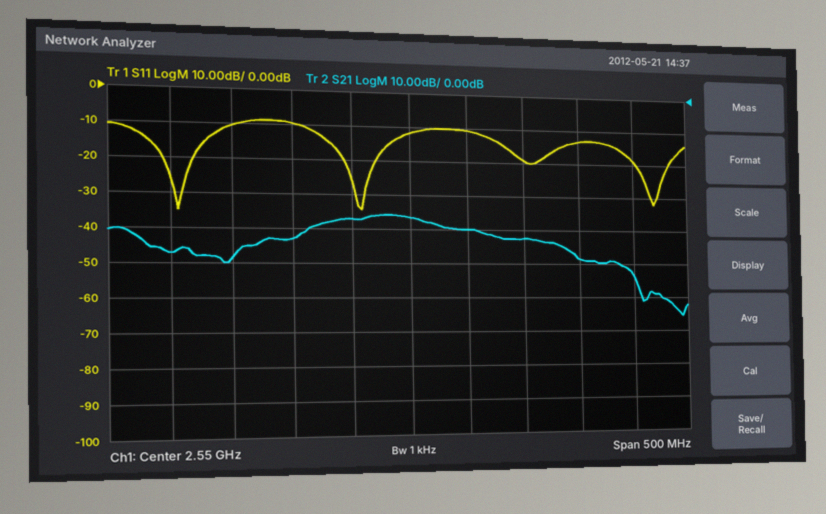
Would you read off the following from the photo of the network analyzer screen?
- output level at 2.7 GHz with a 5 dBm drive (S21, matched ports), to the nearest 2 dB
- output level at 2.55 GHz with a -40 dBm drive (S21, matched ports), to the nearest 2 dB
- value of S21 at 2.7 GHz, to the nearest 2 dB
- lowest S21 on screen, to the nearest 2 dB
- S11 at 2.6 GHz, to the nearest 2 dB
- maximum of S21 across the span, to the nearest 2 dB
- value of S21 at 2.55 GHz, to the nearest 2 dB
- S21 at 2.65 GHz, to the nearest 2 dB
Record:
-44 dBm
-76 dBm
-48 dB
-66 dB
-10 dB
-36 dB
-36 dB
-42 dB
